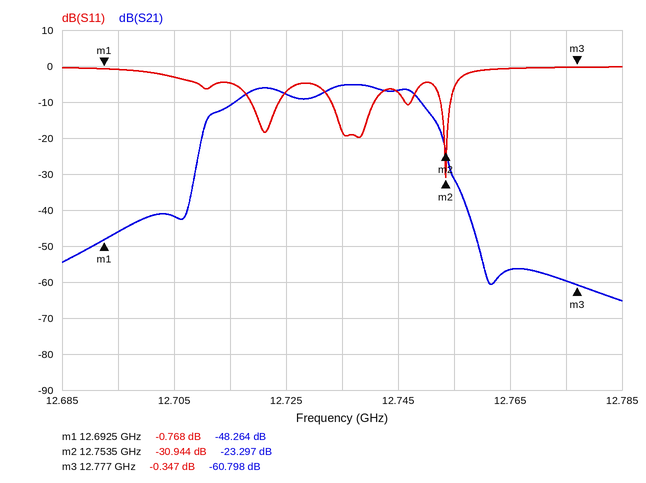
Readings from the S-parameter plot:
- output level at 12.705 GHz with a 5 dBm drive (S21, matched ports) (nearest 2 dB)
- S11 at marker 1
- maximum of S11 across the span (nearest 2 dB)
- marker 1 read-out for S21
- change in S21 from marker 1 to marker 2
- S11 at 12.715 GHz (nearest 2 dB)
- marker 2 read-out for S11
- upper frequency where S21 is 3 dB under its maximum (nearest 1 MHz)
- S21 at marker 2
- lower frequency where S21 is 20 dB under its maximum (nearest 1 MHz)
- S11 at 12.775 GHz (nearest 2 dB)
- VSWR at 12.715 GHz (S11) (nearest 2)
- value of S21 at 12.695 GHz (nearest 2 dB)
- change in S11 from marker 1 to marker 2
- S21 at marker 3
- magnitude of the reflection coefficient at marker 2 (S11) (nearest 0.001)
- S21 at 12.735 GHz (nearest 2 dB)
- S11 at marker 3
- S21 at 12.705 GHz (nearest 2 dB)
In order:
-36 dBm
-0.768 dB
0 dB
-48.264 dB
24.967 dB
-4 dB
-30.944 dB
12.748 GHz
-23.297 dB
12.709 GHz
0 dB
4
-46 dB
-30.176 dB
-60.798 dB
0.028
-6 dB
-0.347 dB
-42 dB
